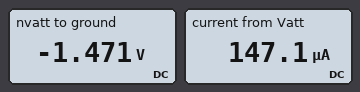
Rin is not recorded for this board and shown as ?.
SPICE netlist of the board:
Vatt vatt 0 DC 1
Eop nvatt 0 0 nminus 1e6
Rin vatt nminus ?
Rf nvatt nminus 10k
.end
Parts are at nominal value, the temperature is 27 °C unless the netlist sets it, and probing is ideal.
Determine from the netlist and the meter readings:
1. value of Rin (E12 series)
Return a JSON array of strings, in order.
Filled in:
["6.8 kΩ"]
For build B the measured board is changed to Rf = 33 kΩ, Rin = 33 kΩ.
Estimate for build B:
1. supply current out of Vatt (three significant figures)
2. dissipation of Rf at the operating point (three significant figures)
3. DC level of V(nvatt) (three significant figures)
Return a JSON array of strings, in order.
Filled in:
["30.3 µA", "30.3 µW", "-1.00 V"]
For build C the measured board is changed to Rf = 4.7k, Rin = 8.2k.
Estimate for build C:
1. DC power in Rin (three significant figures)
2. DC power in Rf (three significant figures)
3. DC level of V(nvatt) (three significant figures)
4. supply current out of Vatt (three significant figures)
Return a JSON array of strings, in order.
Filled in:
["122 µW", "69.9 µW", "-573 mV", "122 µA"]
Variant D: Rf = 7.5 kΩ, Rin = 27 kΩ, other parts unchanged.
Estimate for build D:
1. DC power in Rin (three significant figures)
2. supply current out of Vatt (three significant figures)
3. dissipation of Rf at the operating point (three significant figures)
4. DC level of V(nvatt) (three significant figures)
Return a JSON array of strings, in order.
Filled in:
["37.0 µW", "37.0 µA", "10.3 µW", "-278 mV"]
